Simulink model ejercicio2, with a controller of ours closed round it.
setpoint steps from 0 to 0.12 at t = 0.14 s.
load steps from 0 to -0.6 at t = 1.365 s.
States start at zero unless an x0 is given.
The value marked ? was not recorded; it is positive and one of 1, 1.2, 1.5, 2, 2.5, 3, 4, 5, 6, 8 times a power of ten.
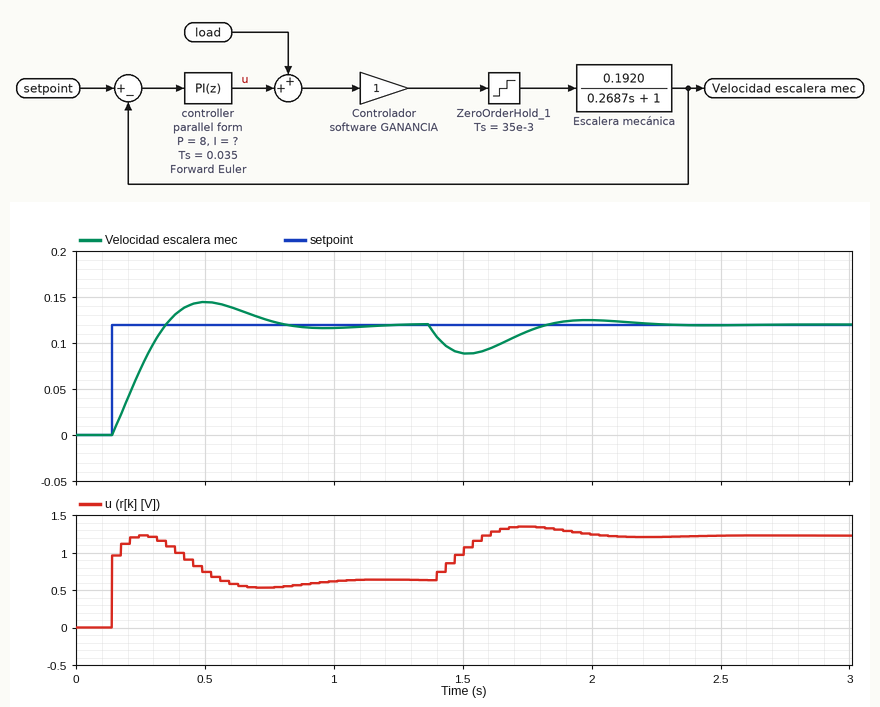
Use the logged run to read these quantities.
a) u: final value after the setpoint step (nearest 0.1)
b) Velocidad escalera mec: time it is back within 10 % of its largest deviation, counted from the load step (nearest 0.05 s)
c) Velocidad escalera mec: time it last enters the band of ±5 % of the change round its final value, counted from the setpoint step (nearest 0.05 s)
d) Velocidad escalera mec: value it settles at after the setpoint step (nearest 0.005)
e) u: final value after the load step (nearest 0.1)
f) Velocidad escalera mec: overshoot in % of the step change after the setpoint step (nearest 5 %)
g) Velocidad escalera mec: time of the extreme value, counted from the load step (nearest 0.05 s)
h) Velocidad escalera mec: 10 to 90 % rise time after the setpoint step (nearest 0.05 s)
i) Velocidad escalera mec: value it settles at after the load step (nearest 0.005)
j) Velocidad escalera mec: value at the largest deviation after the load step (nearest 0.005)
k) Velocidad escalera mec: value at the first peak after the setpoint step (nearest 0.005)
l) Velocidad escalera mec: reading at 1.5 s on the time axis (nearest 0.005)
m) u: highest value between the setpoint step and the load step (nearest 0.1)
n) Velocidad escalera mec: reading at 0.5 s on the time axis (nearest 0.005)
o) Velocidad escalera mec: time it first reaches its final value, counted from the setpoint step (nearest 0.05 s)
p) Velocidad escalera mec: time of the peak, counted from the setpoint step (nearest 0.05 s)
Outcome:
0.6
0.75 s
0.60 s
0.120
1.2
20 %
0.15 s
0.15 s
0.120
0.090
0.145
0.090
1.2
0.145
0.20 s
0.35 s
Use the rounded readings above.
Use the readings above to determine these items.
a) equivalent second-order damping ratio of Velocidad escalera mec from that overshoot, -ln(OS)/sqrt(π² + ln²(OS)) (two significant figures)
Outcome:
0.46
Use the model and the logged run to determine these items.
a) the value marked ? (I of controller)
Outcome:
80
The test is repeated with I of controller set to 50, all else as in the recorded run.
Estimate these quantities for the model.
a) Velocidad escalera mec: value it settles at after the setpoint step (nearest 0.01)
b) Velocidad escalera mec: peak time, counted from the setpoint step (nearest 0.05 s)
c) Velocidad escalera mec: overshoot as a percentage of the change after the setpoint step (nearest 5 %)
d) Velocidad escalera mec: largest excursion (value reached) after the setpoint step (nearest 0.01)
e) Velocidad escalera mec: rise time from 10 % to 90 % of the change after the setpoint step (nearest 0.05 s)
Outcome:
0.12
0.50 s
10 %
0.13
0.20 s
